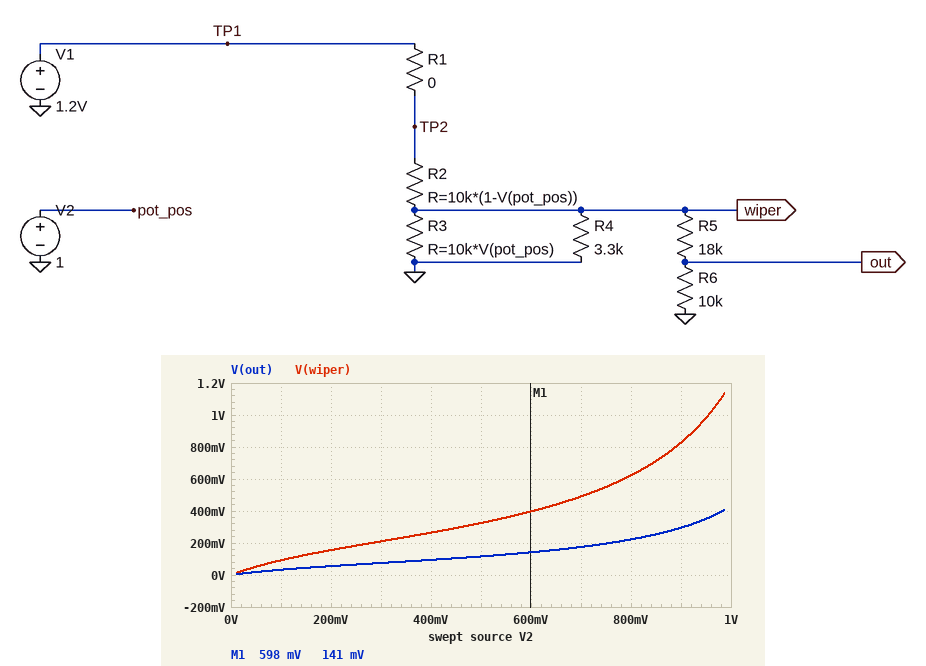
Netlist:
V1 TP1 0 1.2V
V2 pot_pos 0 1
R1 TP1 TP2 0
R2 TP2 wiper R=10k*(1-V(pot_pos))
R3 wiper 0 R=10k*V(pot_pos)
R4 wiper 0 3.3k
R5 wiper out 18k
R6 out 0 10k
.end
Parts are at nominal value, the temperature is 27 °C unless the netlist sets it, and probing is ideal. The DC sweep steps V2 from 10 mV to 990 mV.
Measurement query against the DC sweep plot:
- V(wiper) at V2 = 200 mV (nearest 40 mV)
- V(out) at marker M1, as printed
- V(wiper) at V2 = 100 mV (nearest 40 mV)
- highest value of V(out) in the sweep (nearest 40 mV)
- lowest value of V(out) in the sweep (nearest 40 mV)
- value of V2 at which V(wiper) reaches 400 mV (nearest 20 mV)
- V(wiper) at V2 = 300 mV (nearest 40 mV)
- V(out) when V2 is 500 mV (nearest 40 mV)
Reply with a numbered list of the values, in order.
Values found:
1. 160 mV
2. 141 mV
3. 80 mV
4. 400 mV
5. 0 V
6. 600 mV
7. 200 mV
8. 120 mV
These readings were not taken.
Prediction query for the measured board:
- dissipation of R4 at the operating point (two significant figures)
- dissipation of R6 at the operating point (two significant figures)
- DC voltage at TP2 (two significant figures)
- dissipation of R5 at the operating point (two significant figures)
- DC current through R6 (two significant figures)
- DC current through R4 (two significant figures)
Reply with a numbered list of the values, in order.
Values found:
1. 440 µW
2. 18 µW
3. 1.2 V
4. 33 µW
5. 43 µA
6. 360 µA
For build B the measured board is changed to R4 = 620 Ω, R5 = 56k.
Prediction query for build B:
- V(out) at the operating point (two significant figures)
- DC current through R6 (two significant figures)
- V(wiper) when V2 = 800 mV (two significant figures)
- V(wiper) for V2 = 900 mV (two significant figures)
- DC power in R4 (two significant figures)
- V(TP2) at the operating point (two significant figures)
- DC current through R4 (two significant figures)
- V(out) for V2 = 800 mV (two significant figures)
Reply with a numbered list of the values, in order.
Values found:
1. 180 mV
2. 18 µA
3. 270 mV
4. 440 mV
5. 2.3 mW
6. 1.2 V
7. 1.9 mA
8. 40 mV
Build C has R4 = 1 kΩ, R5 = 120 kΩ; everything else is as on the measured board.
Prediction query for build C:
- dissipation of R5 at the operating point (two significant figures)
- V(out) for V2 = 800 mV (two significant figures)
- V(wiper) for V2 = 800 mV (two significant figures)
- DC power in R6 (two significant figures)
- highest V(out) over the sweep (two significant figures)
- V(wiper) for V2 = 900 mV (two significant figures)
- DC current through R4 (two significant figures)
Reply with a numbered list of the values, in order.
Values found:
1. 10 µW
2. 28 mV
3. 370 mV
4. 850 nW
5. 83 mV
6. 570 mV
7. 1.2 mA
